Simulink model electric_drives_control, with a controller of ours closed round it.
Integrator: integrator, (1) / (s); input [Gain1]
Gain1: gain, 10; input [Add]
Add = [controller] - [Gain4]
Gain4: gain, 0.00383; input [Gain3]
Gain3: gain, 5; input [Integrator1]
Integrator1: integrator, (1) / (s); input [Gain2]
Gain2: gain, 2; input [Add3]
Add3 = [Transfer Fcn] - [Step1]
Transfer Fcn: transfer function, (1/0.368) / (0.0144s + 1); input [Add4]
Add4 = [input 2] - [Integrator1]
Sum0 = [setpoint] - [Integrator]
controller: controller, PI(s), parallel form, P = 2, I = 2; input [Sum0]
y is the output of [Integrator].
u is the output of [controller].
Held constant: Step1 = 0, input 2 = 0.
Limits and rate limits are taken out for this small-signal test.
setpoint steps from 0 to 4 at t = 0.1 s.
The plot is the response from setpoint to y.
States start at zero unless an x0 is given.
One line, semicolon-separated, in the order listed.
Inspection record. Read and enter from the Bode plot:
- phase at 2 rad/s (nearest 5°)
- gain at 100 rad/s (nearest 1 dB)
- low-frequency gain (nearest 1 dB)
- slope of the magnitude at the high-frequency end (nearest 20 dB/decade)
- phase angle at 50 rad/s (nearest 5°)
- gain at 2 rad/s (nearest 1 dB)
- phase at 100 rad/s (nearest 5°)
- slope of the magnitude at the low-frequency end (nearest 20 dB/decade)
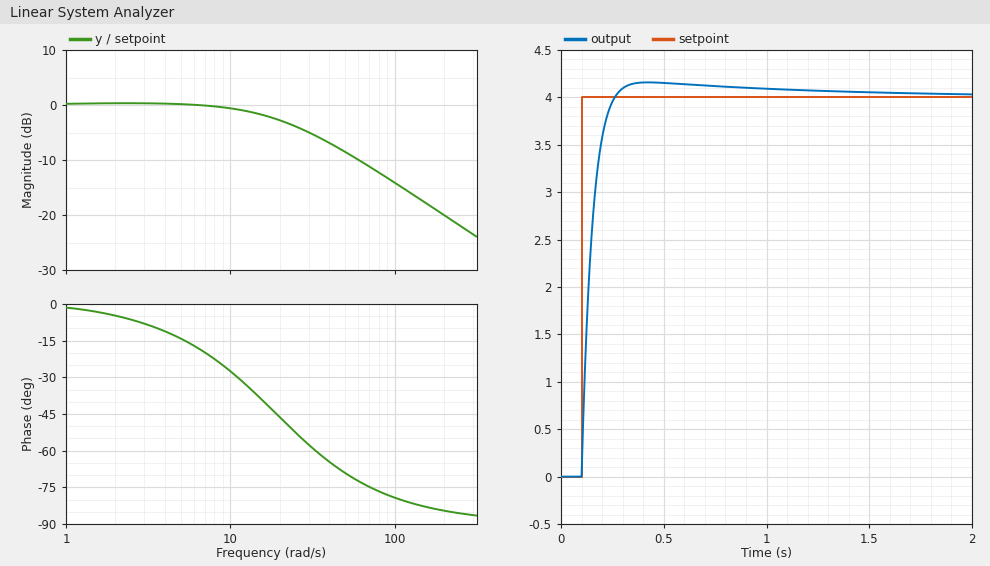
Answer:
-5°; -14 dB; 0 dB; -20 dB/decade; -70°; 0 dB; -80°; 0 dB/decade
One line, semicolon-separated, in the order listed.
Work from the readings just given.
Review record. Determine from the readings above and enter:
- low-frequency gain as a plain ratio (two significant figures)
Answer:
1.0
